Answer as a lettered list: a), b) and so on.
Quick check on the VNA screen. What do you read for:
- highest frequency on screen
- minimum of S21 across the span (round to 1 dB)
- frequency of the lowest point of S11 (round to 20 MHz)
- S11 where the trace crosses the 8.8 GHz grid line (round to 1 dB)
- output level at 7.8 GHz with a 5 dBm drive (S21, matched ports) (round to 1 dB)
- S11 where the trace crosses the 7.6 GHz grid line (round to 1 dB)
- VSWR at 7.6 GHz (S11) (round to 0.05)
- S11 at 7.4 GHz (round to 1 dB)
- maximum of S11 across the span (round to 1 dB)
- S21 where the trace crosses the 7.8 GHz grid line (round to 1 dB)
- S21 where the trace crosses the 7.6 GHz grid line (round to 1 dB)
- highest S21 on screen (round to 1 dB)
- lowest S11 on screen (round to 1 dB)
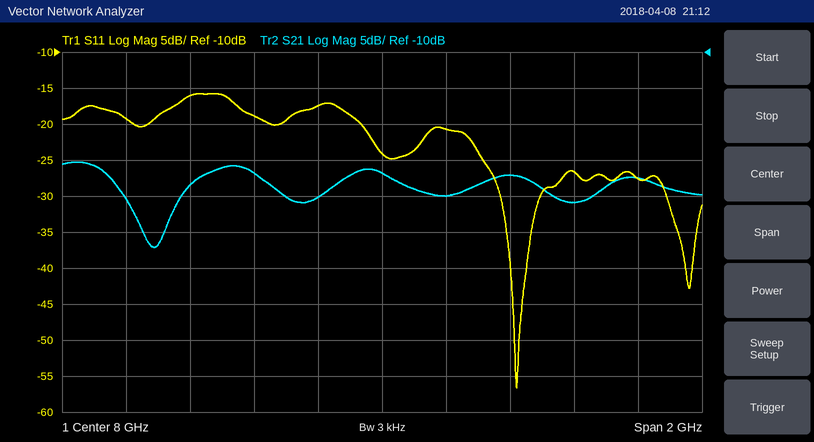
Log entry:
a) 9 GHz
b) -37 dB
c) 8.42 GHz
d) -28 dB
e) -25 dBm
f) -19 dB
g) 1.25
h) -16 dB
i) -16 dB
j) -30 dB
k) -27 dB
l) -25 dB
m) -57 dB
